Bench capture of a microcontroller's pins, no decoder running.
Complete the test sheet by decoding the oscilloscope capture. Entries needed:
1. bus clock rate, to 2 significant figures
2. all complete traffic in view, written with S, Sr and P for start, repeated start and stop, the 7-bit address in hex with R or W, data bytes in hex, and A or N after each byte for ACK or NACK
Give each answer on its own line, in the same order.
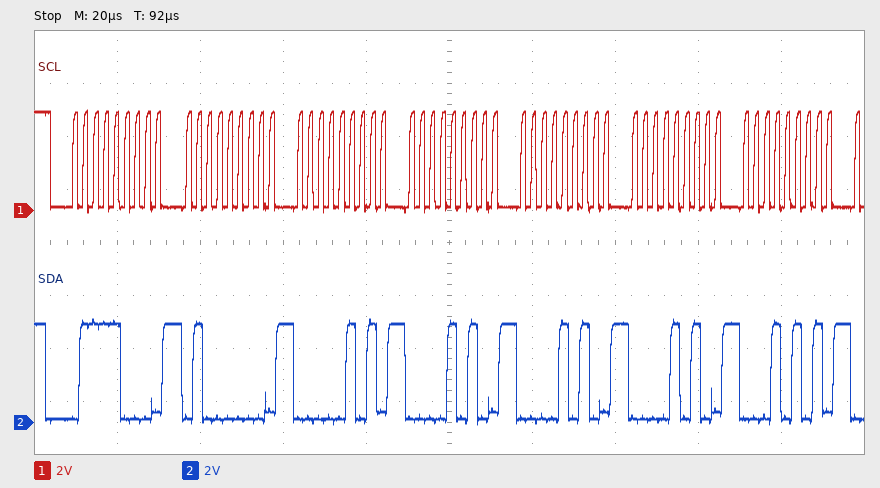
400 kHz
S 3CW A 40 A 05 A 0A A 0A A 0A A 15 A
